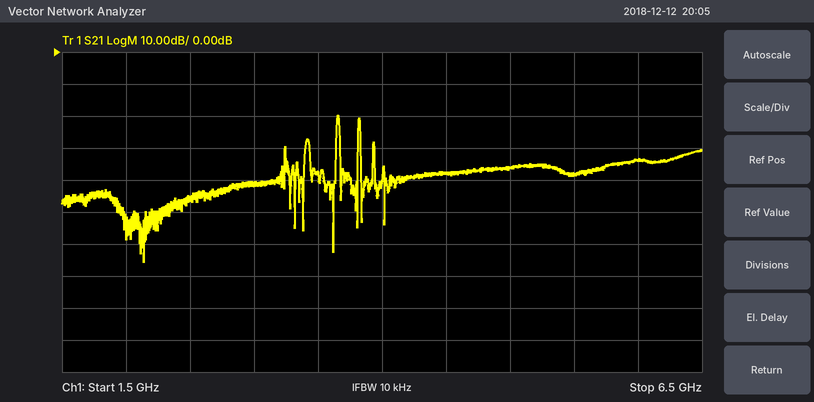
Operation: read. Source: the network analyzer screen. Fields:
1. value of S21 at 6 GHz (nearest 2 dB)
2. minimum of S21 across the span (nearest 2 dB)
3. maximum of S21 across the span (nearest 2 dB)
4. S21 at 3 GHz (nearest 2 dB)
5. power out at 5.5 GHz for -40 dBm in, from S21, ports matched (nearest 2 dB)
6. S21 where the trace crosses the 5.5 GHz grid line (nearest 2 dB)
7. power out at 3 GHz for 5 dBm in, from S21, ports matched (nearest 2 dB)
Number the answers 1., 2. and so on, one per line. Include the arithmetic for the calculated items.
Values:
1. -34 dB
2. -66 dB
3. -20 dB
4. -42 dB
5. -40 dBm + (-38 dB) = -78 dBm
6. -38 dB
7. 5 dBm + (-42 dB) = -36 dBm
